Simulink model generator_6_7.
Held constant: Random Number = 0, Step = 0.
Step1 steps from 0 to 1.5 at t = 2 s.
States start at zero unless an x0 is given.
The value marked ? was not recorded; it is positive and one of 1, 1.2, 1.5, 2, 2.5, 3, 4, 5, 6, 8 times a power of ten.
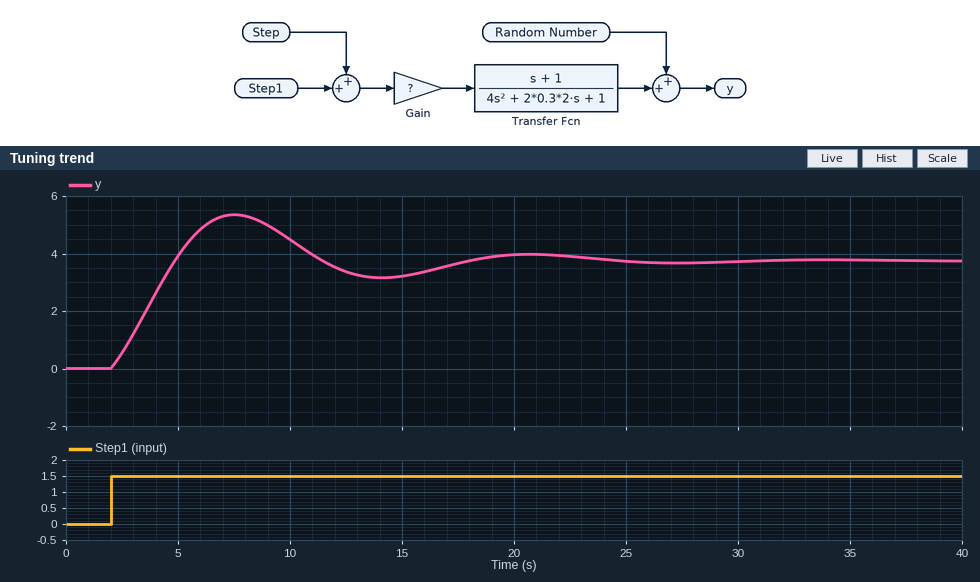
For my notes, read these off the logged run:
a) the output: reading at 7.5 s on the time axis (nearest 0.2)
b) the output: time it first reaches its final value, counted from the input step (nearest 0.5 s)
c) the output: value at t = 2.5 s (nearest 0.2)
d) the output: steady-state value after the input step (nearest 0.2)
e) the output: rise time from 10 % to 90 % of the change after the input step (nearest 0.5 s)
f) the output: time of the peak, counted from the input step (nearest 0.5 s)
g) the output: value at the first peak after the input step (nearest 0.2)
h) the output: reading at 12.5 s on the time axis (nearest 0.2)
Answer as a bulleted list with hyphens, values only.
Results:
- 5.4
- 3.0 s
- 0.6
- 3.8
- 2.0 s
- 5.5 s
- 5.4
- 3.4
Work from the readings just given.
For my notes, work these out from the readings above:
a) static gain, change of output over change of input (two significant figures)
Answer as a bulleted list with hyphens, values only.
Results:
- 2.5
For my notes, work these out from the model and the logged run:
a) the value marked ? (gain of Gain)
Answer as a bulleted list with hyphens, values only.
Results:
- 2.5
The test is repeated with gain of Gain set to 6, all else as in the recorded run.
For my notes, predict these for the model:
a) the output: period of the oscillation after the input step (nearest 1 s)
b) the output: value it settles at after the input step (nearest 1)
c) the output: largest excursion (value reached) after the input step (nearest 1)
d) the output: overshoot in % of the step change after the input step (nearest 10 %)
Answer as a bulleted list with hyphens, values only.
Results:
- 13 s
- 9
- 13
- 40 %
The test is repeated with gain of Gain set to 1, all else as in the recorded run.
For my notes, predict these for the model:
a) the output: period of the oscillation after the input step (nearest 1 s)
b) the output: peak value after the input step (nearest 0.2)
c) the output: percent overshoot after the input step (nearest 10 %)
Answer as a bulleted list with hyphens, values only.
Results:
- 13 s
- 2.2
- 40 %
